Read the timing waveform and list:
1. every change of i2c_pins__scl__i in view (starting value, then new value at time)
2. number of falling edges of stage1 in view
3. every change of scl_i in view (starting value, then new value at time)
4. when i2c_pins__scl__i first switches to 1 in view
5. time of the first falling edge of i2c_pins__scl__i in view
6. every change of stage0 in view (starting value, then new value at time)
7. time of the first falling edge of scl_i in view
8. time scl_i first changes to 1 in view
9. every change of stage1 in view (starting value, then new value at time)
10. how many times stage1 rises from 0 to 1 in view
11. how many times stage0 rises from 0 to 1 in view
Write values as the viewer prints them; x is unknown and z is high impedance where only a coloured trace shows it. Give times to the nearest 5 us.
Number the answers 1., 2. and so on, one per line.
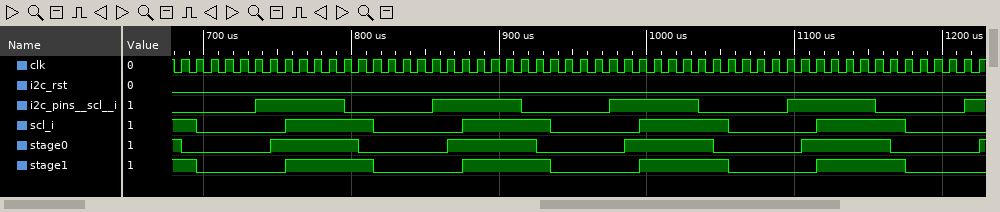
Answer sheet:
1. 0, 1 at 735 us, 0 at 795 us, 1 at 855 us, 0 at 915 us, 1 at 975 us, 0 at 1035 us, 1 at 1095 us, 0 at 1155 us, 1 at 1215 us
2. 5
3. 1, 0 at 695 us, 1 at 755 us, 0 at 815 us, 1 at 875 us, 0 at 935 us, 1 at 995 us, 0 at 1055 us, 1 at 1115 us, 0 at 1175 us
4. 735 us
5. 795 us
6. 1, 0 at 685 us, 1 at 745 us, 0 at 805 us, 1 at 865 us, 0 at 925 us, 1 at 985 us, 0 at 1045 us, 1 at 1105 us, 0 at 1165 us, 1 at 1225 us
7. 695 us
8. 755 us
9. 1, 0 at 695 us, 1 at 755 us, 0 at 815 us, 1 at 875 us, 0 at 935 us, 1 at 995 us, 0 at 1055 us, 1 at 1115 us, 0 at 1175 us
10. 4
11. 5
